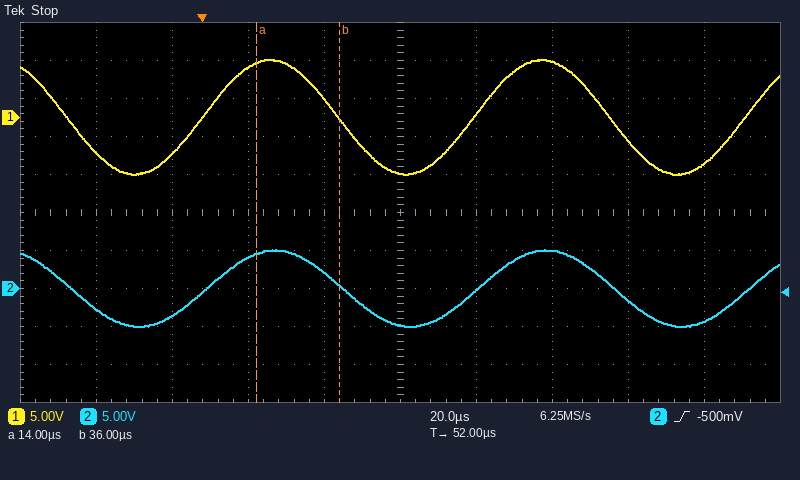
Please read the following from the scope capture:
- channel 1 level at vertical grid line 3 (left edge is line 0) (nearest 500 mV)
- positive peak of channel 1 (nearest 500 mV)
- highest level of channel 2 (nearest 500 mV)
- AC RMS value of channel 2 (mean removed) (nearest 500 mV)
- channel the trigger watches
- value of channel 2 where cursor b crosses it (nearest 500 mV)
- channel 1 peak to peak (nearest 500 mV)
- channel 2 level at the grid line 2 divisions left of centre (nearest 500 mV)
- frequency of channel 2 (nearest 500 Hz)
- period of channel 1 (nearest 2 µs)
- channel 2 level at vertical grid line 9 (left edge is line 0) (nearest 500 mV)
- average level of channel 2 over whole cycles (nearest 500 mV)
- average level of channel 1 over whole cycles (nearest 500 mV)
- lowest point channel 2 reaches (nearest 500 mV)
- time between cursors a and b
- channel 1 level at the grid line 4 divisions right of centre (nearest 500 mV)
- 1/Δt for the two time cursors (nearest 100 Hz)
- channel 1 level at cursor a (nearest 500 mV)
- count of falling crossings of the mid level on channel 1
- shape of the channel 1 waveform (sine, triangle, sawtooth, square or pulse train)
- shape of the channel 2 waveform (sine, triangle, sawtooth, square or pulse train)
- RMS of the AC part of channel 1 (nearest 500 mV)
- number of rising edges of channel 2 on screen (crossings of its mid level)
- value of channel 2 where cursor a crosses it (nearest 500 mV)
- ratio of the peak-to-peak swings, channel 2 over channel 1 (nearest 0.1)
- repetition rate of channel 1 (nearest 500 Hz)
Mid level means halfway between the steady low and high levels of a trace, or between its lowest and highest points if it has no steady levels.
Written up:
6.5 V
7.5 V
5.0 V
3.5 V
channel 2
500 mV
15.0 V
4.0 V
14.0 kHz
72 µs
-4.5 V
0.0 V
0.0 V
-5.0 V
22 µs
-6.0 V
45.5 kHz
7.0 V
3
sine
sine
5.5 V
3
4.5 V
0.7
14.0 kHz
